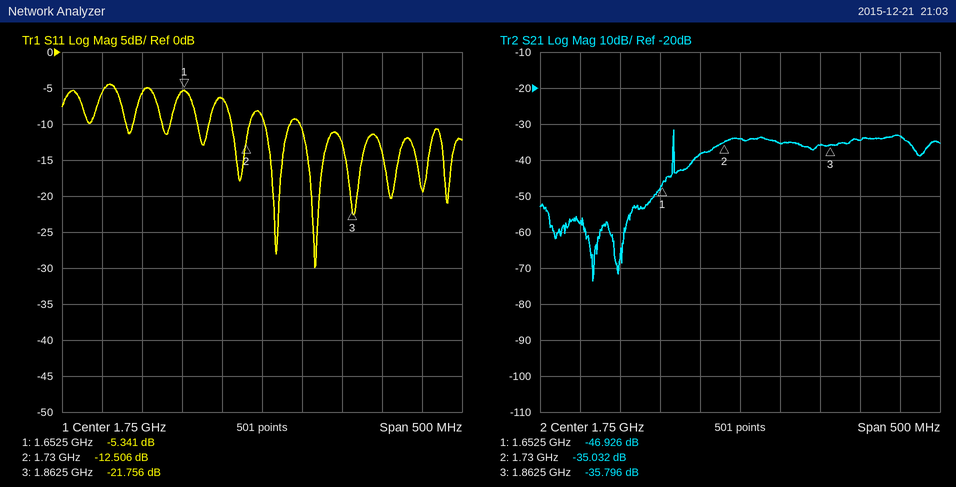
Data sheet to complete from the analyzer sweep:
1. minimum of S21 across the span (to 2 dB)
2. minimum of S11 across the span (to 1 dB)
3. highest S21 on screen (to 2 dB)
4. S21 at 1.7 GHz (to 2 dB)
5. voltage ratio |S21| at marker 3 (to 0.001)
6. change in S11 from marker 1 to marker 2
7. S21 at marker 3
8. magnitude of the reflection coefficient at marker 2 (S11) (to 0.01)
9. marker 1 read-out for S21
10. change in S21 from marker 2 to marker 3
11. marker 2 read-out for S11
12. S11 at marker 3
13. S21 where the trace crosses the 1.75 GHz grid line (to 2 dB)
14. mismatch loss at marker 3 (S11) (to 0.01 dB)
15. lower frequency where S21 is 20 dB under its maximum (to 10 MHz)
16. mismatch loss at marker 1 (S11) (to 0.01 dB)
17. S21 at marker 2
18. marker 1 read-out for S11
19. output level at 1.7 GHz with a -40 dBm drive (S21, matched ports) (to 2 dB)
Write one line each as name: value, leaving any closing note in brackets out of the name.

minimum of S21 across the span: -74 dB
minimum of S11 across the span: -30 dB
highest S21 on screen: -32 dB
S21 at 1.7 GHz: -38 dB
voltage ratio |S21| at marker 3: 0.016
change in S11 from marker 1 to marker 2: -7.165 dB
S21 at marker 3: -35.796 dB
magnitude of the reflection coefficient at marker 2 (S11): 0.24
marker 1 read-out for S21: -46.926 dB
change in S21 from marker 2 to marker 3: -0.764 dB
marker 2 read-out for S11: -12.506 dB
S11 at marker 3: -21.756 dB
S21 where the trace crosses the 1.75 GHz grid line: -34 dB
mismatch loss at marker 3 (S11): 0.03 dB
lower frequency where S21 is 20 dB under its maximum: 1.64 GHz
mismatch loss at marker 1 (S11): 1.50 dB
S21 at marker 2: -35.032 dB
marker 1 read-out for S11: -5.341 dB
output level at 1.7 GHz with a -40 dBm drive (S21, matched ports): -78 dBm
